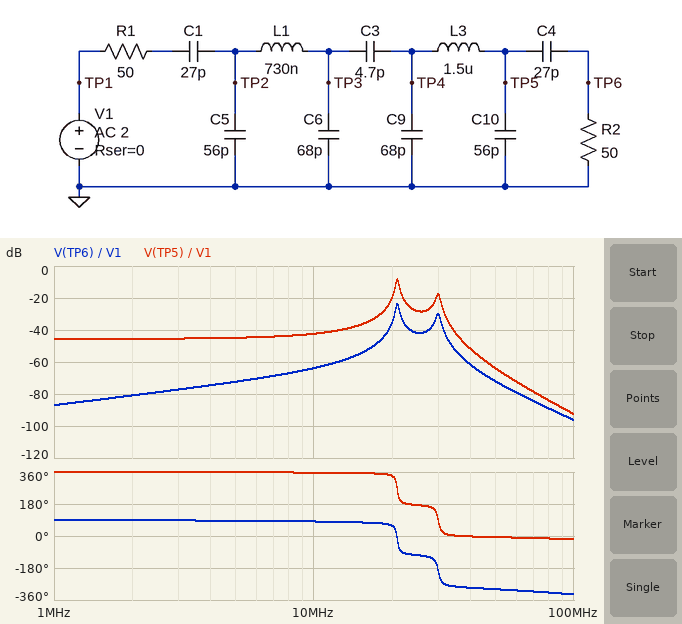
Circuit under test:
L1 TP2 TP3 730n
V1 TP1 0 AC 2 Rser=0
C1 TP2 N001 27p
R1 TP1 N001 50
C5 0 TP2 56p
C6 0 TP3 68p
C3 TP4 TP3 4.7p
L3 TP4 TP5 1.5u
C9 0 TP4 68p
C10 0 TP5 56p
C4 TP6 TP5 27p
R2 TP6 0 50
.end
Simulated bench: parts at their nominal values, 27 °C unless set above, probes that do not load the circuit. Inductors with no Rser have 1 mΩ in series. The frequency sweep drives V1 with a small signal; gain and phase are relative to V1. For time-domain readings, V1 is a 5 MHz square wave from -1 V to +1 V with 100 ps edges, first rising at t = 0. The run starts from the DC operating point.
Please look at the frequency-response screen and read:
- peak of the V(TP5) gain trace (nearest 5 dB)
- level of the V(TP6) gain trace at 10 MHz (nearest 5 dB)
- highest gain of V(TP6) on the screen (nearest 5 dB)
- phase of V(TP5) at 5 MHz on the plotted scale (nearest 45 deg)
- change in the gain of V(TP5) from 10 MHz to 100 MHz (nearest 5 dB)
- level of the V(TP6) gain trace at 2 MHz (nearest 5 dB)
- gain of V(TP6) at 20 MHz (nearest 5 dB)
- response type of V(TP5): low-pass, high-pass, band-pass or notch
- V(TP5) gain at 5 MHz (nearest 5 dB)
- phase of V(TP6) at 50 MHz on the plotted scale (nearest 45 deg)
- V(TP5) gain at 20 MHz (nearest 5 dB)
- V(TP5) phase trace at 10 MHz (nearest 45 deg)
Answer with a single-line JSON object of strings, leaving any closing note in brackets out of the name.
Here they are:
{"peak of the V(TP5) gain trace": "-10 dB", "level of the V(TP6) gain trace at 10 MHz": "-65 dB", "highest gain of V(TP6) on the screen": "-25 dB", "phase of V(TP5) at 5 MHz on the plotted scale": "360 deg", "change in the gain of V(TP5) from 10 MHz to 100 MHz": "-50 dB", "level of the V(TP6) gain trace at 2 MHz": "-80 dB", "gain of V(TP6) at 20 MHz": "-35 dB", "response type of V(TP5): low-pass, high-pass, band-pass or notch": "band-pass", "V(TP5) gain at 5 MHz": "-45 dB", "phase of V(TP6) at 50 MHz on the plotted scale": "-315 deg", "V(TP5) gain at 20 MHz": "-20 dB", "V(TP5) phase trace at 10 MHz": "360 deg"}
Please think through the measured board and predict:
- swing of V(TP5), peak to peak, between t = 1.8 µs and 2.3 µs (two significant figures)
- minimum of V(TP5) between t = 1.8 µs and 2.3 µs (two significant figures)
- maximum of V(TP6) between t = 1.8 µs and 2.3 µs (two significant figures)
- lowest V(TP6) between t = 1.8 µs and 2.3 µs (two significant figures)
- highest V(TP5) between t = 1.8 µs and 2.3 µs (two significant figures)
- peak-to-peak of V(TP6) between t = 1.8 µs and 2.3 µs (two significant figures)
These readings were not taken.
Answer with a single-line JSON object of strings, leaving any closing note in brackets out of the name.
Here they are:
{"swing of V(TP5), peak to peak, between t = 1.8 µs and 2.3 µs": "38 mV", "minimum of V(TP5) between t = 1.8 µs and 2.3 µs": "-13 mV", "maximum of V(TP6) between t = 1.8 µs and 2.3 µs": "2.9 mV", "lowest V(TP6) between t = 1.8 µs and 2.3 µs": "-3.0 mV", "highest V(TP5) between t = 1.8 µs and 2.3 µs": "24 mV", "peak-to-peak of V(TP6) between t = 1.8 µs and 2.3 µs": "6.0 mV"}
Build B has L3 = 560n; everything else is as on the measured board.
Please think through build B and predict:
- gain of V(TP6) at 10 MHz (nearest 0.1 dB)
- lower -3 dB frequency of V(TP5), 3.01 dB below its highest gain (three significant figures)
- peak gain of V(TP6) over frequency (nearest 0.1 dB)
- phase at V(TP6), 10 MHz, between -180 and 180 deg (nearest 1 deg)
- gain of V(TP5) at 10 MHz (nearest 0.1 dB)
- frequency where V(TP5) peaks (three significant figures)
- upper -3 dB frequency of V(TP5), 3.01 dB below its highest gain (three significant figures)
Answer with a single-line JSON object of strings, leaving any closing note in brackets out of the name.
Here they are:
{"gain of V(TP6) at 10 MHz": "-65.3 dB", "lower -3 dB frequency of V(TP5), 3.01 dB below its highest gain": "29.5 MHz", "peak gain of V(TP6) over frequency": "-17.0 dB", "phase at V(TP6), 10 MHz, between -180 and 180 deg": "82 deg", "gain of V(TP5) at 10 MHz": "-43.8 dB", "frequency where V(TP5) peaks": "30.0 MHz", "upper -3 dB frequency of V(TP5), 3.01 dB below its highest gain": "30.7 MHz"}
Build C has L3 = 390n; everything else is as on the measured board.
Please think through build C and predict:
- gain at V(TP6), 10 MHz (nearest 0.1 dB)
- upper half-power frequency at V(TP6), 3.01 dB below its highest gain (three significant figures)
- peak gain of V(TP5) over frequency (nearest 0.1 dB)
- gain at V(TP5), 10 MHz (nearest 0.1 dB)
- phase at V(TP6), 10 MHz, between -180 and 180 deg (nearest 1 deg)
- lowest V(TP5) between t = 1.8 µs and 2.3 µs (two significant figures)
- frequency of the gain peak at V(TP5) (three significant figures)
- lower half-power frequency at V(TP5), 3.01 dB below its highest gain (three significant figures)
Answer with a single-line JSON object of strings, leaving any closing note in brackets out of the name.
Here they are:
{"gain at V(TP6), 10 MHz": "-65.5 dB", "upper half-power frequency at V(TP6), 3.01 dB below its highest gain": "30.6 MHz", "peak gain of V(TP5) over frequency": "-10.6 dB", "gain at V(TP5), 10 MHz": "-44.1 dB", "phase at V(TP6), 10 MHz, between -180 and 180 deg": "82 deg", "lowest V(TP5) between t = 1.8 µs and 2.3 µs": "-17 mV", "frequency of the gain peak at V(TP5)": "30.0 MHz", "lower half-power frequency at V(TP5), 3.01 dB below its highest gain": "29.5 MHz"}
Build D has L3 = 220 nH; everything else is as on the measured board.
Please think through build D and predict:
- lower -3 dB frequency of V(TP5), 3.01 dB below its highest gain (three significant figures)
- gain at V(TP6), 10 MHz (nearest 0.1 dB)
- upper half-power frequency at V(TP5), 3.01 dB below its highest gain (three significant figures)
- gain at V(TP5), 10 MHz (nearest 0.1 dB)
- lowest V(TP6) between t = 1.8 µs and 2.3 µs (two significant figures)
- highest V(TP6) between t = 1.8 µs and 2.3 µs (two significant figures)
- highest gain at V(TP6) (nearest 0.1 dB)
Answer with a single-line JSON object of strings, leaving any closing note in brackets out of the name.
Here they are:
{"lower -3 dB frequency of V(TP5), 3.01 dB below its highest gain": "29.5 MHz", "gain at V(TP6), 10 MHz": "-65.8 dB", "upper half-power frequency at V(TP5), 3.01 dB below its highest gain": "30.6 MHz", "gain at V(TP5), 10 MHz": "-44.3 dB", "lowest V(TP6) between t = 1.8 µs and 2.3 µs": "-4.0 mV", "highest V(TP6) between t = 1.8 µs and 2.3 µs": "4.0 mV", "highest gain at V(TP6)": "-26.2 dB"}
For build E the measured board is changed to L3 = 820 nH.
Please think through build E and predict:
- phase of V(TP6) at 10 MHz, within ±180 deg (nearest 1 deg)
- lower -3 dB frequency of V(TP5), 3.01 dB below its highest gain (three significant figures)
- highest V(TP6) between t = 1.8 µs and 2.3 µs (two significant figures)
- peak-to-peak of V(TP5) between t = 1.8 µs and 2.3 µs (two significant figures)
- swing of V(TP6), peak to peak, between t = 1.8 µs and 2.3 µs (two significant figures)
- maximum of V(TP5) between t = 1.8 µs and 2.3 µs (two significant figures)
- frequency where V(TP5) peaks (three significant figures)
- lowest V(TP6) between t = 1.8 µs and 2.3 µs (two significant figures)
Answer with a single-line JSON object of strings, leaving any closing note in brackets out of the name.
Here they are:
{"phase of V(TP6) at 10 MHz, within ±180 deg": "82 deg", "lower -3 dB frequency of V(TP5), 3.01 dB below its highest gain": "27.9 MHz", "highest V(TP6) between t = 1.8 µs and 2.3 µs": "6.4 mV", "peak-to-peak of V(TP5) between t = 1.8 µs and 2.3 µs": "60 mV", "swing of V(TP6), peak to peak, between t = 1.8 µs and 2.3 µs": "13 mV", "maximum of V(TP5) between t = 1.8 µs and 2.3 µs": "35 mV", "frequency where V(TP5) peaks": "28.3 MHz", "lowest V(TP6) between t = 1.8 µs and 2.3 µs": "-6.4 mV"}
